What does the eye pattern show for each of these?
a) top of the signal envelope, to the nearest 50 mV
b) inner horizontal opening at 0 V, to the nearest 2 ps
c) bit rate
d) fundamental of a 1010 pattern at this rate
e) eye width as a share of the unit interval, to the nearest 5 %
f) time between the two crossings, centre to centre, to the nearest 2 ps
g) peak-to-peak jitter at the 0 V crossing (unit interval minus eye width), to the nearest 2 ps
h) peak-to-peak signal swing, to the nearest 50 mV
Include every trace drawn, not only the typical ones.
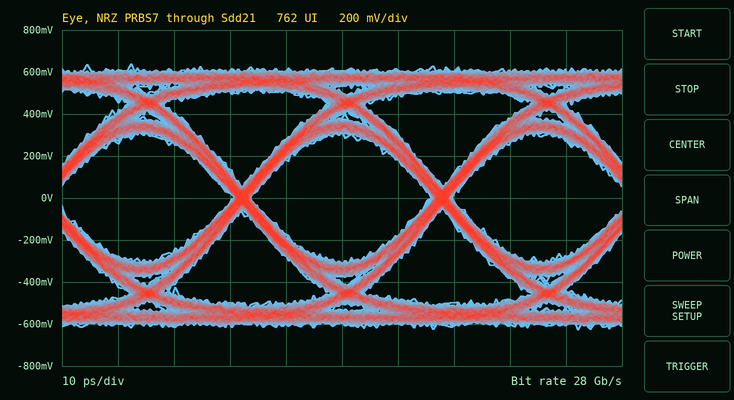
650 mV
32 ps
28 Gb/s
14 GHz
90 %
36 ps
4 ps
1.25 V
